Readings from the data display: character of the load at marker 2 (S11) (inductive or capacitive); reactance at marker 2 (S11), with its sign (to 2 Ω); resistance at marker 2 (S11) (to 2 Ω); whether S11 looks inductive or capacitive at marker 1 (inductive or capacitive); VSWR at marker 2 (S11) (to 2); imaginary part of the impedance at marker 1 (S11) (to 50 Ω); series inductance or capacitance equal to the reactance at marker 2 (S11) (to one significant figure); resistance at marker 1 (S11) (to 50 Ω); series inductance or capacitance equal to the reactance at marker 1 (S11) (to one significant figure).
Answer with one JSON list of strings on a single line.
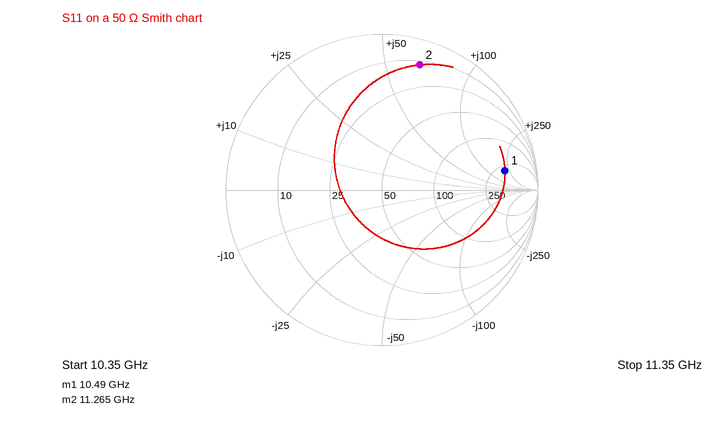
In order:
["inductive", "+66 Ω", "12 Ω", "inductive", "12", "+200 Ω", "900 pH", "300 Ω", "3 nH"]
